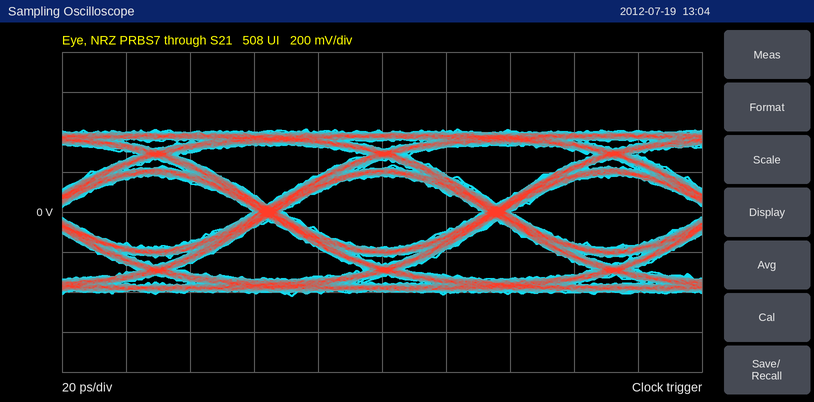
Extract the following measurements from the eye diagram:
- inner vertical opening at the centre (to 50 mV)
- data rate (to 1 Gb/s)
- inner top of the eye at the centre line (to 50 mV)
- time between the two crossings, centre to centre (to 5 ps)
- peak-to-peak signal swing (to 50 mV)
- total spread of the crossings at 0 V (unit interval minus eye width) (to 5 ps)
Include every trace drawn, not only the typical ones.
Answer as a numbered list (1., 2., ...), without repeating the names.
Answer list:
1. 350 mV
2. 14 Gb/s
3. 200 mV
4. 70 ps
5. 850 mV
6. 10 ps
